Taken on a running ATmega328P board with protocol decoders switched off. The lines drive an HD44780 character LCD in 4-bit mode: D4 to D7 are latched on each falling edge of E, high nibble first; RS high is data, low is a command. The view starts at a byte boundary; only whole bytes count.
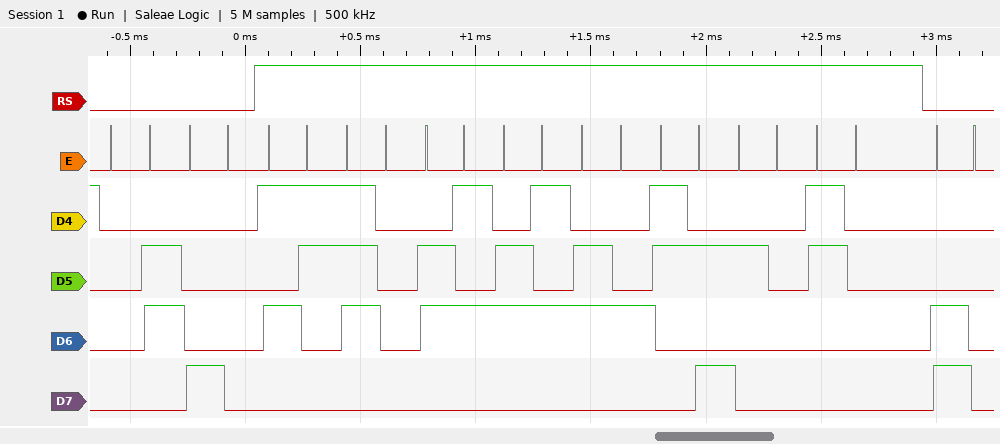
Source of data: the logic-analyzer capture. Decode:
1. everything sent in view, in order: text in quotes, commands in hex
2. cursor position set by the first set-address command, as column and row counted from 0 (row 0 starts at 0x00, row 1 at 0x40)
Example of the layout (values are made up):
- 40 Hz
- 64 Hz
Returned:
- 0x06 0x80 "Speed: 0" 0xC0
- column 0, row 0
